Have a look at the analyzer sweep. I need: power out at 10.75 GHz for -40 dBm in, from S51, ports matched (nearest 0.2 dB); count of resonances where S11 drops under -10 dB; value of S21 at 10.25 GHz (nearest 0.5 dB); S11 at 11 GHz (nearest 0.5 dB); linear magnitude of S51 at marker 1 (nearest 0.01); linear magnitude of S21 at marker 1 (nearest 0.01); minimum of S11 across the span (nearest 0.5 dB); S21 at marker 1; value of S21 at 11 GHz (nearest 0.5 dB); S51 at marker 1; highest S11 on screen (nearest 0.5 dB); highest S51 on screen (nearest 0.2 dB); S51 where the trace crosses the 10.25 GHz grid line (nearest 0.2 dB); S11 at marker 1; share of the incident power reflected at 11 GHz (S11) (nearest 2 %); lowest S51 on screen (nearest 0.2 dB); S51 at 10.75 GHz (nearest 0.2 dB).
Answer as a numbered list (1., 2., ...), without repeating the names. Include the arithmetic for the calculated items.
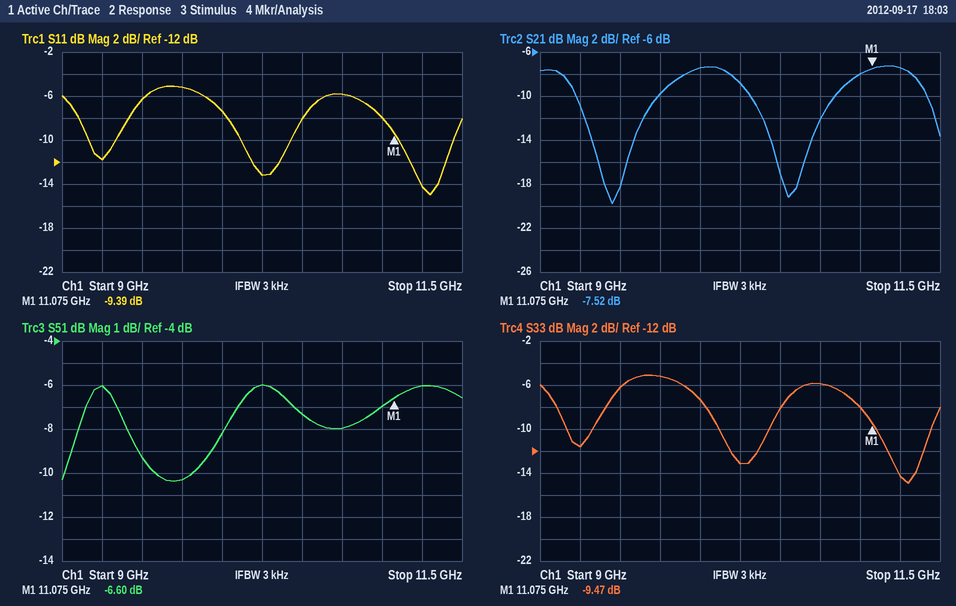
1. -40 dBm + (-8.0 dB) = -48.0 dBm
2. 3
3. -9.0 dB
4. -8.0 dB
5. 10^(-6.6/20) ≈ 0.47
6. 10^(-7.52/20) ≈ 0.42
7. -15.0 dB
8. -7.52 dB
9. -8.0 dB
10. -6.60 dB
11. -5.0 dB
12. -6.0 dB
13. -6.0 dB
14. -9.39 dB
15. 10^(-8/10) ≈ 16 %
16. -10.4 dB
17. -8.0 dB
